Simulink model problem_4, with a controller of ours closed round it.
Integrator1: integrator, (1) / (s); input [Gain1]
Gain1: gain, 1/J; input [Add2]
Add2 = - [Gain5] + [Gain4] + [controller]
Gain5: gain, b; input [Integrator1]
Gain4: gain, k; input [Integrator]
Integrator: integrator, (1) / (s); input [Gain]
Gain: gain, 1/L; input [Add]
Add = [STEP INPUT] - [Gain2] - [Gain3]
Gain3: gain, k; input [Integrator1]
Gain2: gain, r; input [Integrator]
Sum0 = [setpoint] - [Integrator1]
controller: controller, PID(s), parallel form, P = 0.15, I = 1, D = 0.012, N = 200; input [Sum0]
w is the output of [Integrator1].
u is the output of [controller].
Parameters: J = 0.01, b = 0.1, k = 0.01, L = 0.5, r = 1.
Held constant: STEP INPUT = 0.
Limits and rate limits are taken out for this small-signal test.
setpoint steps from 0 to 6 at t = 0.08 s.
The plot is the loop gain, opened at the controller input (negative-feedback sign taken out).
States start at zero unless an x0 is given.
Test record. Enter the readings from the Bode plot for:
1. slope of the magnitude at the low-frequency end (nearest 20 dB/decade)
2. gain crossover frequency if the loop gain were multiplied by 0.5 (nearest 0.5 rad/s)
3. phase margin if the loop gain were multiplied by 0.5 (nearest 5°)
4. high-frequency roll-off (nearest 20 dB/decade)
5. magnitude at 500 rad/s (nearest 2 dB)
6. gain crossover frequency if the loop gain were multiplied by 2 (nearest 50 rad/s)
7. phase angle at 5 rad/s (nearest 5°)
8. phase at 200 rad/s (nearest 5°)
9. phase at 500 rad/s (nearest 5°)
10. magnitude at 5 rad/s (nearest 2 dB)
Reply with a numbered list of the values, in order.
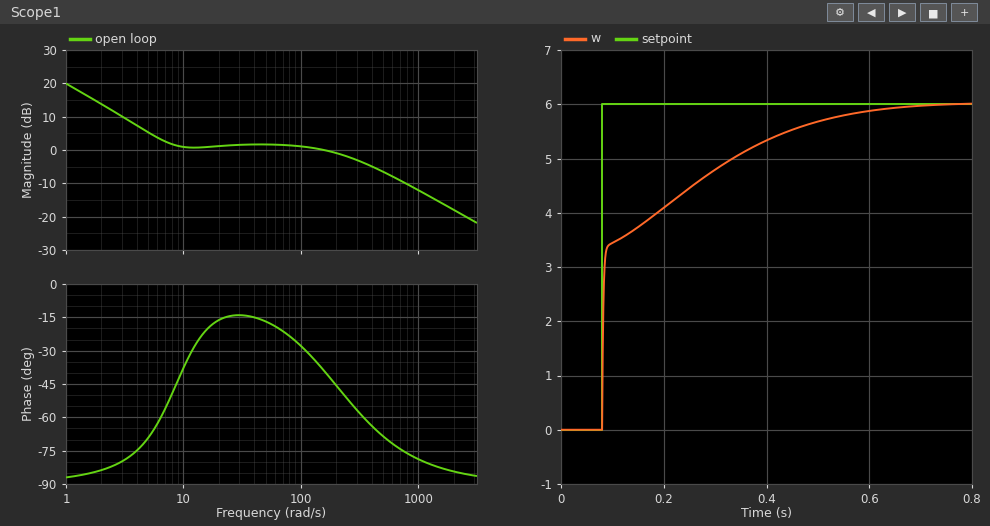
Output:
1. -20 dB/decade
2. 4.5 rad/s
3. 110°
4. -20 dB/decade
5. -6 dB
6. 450 rad/s
7. -70°
8. -45°
9. -70°
10. 6 dB
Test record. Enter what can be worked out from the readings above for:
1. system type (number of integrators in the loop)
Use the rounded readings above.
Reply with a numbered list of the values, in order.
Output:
1. 1
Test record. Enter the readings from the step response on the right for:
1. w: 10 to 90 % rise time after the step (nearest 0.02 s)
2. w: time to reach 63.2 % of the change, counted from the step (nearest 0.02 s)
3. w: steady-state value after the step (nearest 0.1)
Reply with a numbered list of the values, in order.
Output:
1. 0.34 s
2. 0.08 s
3. 6.0
